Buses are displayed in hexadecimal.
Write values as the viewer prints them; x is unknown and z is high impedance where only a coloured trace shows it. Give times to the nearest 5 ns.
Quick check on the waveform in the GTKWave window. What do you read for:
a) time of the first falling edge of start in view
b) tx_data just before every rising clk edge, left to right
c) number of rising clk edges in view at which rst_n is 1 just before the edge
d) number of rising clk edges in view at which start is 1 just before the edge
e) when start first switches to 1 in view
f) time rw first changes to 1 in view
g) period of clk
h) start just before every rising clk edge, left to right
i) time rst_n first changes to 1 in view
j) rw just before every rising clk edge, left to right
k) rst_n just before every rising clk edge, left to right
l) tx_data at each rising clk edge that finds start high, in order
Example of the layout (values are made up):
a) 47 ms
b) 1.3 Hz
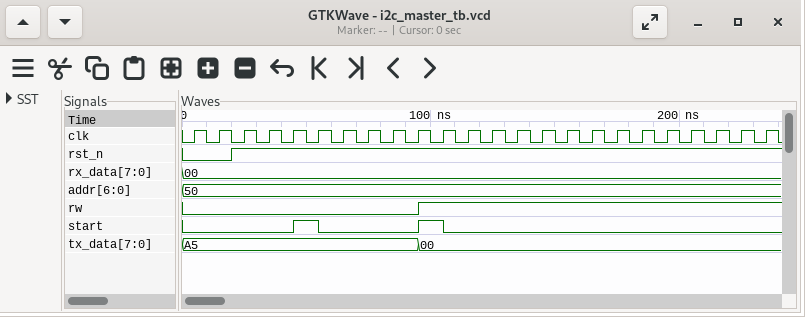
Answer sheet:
a) 55 ns
b) A5, A5, A5, A5, A5, A5, A5, A5, A5, A5, 00, 00, 00, 00, 00, 00, 00, 00, 00, 00, 00, 00, 00, 00
c) 22
d) 2
e) 45 ns
f) 95 ns
g) 10 ns
h) 0 0 0 0 0 1 0 0 0 0 1 0 0 0 0 0 0 0 0 0 0 0 0 0
i) 20 ns
j) 0 0 0 0 0 0 0 0 0 0 1 1 1 1 1 1 1 1 1 1 1 1 1 1
k) 0 0 1 1 1 1 1 1 1 1 1 1 1 1 1 1 1 1 1 1 1 1 1 1
l) A5, 00
